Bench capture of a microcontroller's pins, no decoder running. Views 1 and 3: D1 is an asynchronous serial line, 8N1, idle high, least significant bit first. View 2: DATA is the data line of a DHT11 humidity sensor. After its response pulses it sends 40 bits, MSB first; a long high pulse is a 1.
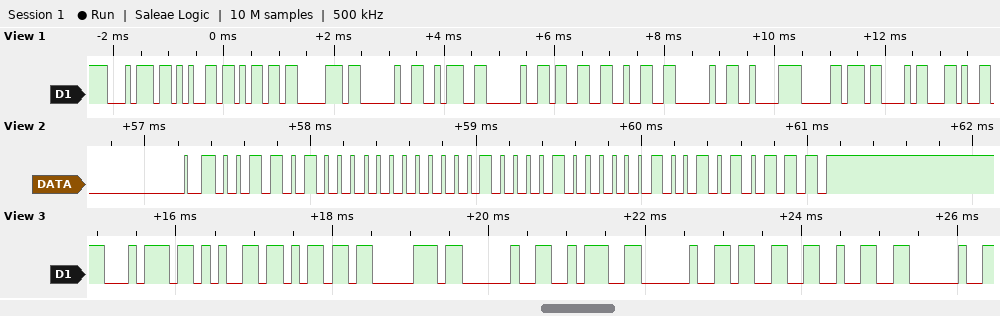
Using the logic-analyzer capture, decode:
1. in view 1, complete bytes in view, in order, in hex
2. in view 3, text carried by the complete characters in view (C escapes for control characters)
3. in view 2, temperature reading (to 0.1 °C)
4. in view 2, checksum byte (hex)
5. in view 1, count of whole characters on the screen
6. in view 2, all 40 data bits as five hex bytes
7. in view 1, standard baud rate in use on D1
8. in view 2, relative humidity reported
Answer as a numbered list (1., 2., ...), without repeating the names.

1. 74 65 6D 70 20 3A 20 33 32 20 C2 B0 43 2C
2. "temp : 32 "
3. 33.2 °C
4. 0x57
5. 14
6. 34 00 21 02 57
7. 9600 baud
8. 52 %
